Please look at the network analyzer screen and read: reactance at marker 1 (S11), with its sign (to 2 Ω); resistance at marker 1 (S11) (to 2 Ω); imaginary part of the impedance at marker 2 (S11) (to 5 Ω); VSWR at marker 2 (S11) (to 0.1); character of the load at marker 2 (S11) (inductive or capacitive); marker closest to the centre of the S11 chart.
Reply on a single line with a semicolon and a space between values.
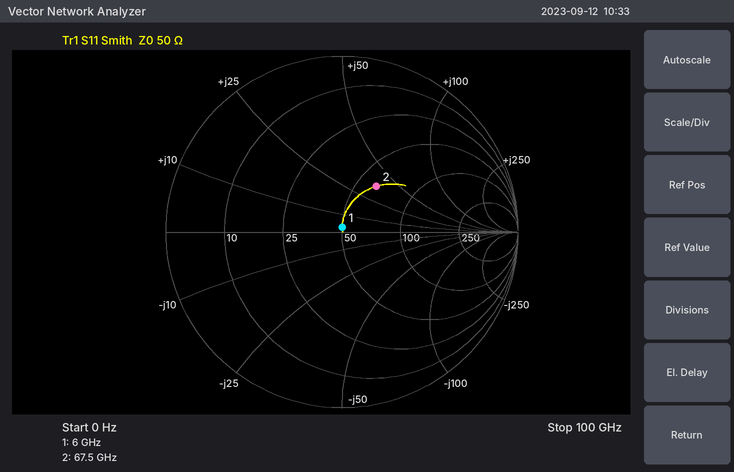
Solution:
+2 Ω; 50 Ω; +35 Ω; 2.0; inductive; marker 1
